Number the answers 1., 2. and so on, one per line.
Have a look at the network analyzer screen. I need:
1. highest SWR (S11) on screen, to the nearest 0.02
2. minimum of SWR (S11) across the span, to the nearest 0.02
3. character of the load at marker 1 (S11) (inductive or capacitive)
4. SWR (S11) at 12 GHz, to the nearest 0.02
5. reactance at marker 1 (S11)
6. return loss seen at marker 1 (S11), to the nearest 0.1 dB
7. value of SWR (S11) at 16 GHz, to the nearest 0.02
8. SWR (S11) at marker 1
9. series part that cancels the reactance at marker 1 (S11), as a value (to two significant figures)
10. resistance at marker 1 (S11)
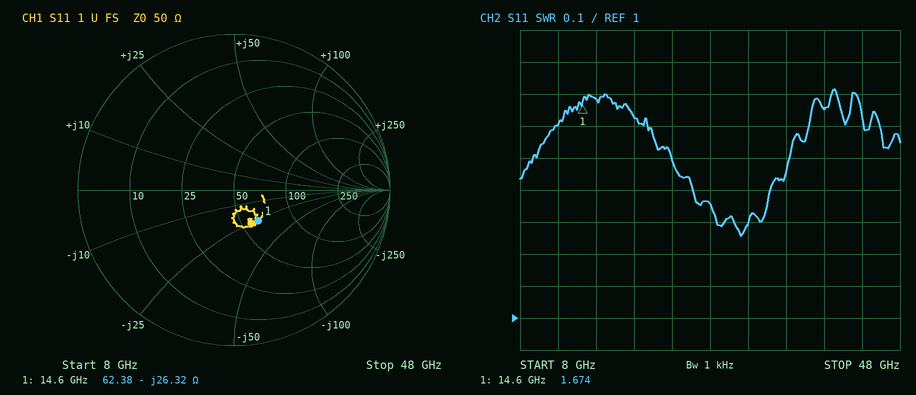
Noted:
1. 1.72
2. 1.26
3. capacitive
4. 1.60
5. -26.32 Ω
6. 12.0 dB
7. 1.68
8. 1.674
9. 290 pH
10. 62.38 Ω
